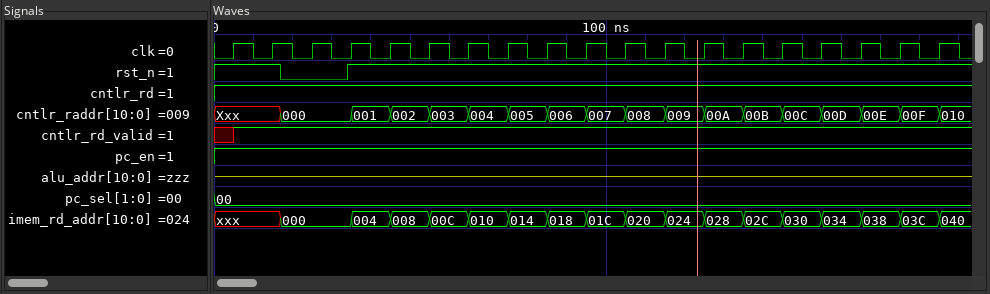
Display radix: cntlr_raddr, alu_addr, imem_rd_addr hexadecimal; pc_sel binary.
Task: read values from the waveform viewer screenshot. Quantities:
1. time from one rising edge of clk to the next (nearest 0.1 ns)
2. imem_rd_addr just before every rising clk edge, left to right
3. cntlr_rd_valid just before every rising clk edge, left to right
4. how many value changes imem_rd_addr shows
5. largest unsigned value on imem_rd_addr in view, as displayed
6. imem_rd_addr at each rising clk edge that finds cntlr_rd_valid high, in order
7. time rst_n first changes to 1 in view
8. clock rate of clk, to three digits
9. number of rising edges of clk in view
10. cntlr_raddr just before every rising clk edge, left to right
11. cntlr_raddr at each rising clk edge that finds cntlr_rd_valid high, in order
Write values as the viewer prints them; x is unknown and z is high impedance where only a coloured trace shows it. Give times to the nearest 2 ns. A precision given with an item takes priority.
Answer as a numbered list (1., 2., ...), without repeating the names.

1. 10 ns
2. xxx, xxx, 000, 000, 004, 008, 00C, 010, 014, 018, 01C, 020, 024, 028, 02C, 030, 034, 038, 03C
3. x 1 1 1 1 1 1 1 1 1 1 1 1 1 1 1 1 1 1
4. 17
5. 040
6. xxx, 000, 000, 004, 008, 00C, 010, 014, 018, 01C, 020, 024, 028, 02C, 030, 034, 038, 03C
7. 34 ns
8. 100 MHz
9. 19
10. Xxx, Xxx, 000, 000, 001, 002, 003, 004, 005, 006, 007, 008, 009, 00A, 00B, 00C, 00D, 00E, 00F
11. Xxx, 000, 000, 001, 002, 003, 004, 005, 006, 007, 008, 009, 00A, 00B, 00C, 00D, 00E, 00F
